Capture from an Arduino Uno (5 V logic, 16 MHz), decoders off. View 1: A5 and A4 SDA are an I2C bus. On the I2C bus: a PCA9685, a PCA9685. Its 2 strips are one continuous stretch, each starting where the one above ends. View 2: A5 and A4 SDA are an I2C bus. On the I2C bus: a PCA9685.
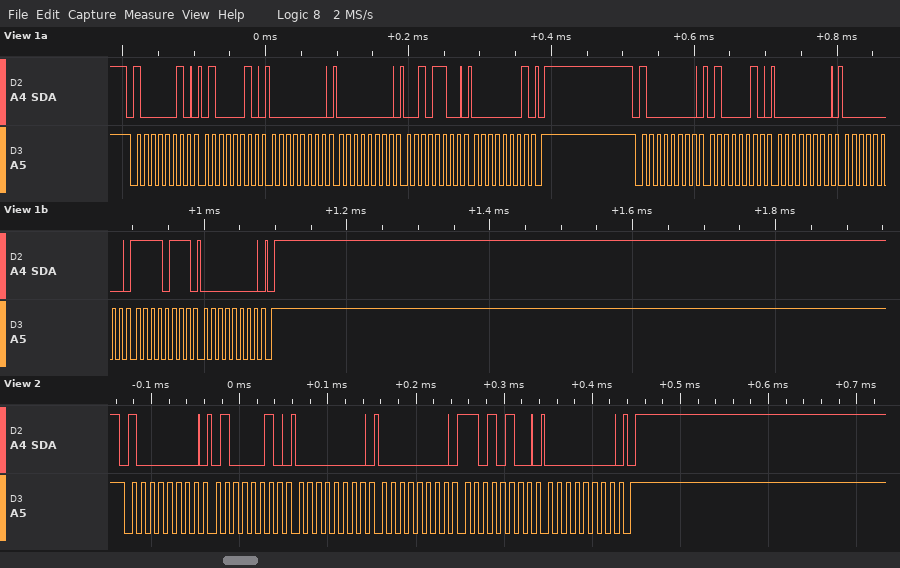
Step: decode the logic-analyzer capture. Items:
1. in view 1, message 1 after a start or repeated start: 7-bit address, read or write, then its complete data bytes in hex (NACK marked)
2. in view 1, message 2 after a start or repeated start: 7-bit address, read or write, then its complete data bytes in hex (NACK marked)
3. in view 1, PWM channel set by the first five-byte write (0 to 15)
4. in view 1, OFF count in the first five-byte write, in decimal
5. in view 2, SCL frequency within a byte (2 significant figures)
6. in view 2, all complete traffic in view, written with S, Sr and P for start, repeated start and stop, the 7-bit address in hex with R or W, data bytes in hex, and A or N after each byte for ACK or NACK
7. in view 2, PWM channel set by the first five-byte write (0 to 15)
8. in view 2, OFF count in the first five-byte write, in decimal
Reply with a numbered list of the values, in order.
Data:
1. 0x41 write: 42 00 00 2C 01
2. 0x40 write: 42 00 00 F7 00
3. 15
4. 300
5. 100 kHz
6. S 40W A 42 A 00 A 00 A D4 A 00 A P
7. 15
8. 212
